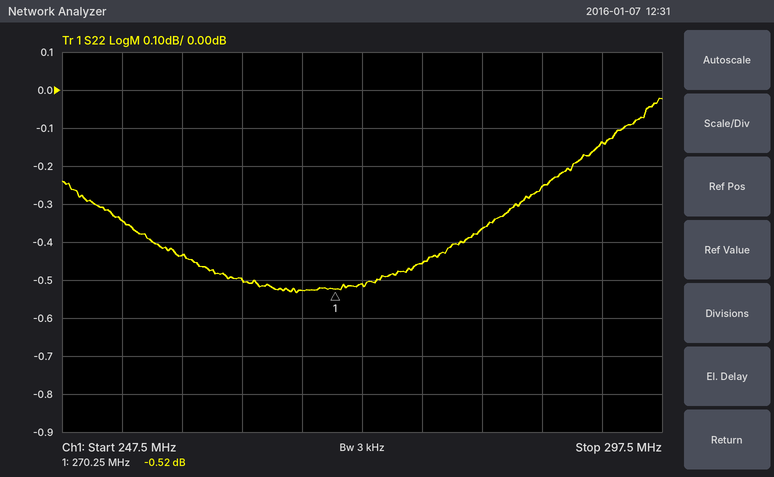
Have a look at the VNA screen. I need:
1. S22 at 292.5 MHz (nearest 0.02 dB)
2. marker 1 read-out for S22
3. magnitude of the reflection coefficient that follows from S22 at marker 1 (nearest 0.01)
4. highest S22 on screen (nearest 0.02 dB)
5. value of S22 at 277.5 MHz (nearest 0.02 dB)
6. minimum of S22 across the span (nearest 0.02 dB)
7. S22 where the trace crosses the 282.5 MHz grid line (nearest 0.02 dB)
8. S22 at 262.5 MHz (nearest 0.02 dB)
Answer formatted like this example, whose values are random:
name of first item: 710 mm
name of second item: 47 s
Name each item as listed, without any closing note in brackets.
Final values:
S22 at 292.5 MHz: -0.14 dB
marker 1 read-out for S22: -0.52 dB
magnitude of the reflection coefficient that follows from S22 at marker 1: 0.94
highest S22 on screen: -0.02 dB
value of S22 at 277.5 MHz: -0.46 dB
minimum of S22 across the span: -0.54 dB
S22 where the trace crosses the 282.5 MHz grid line: -0.36 dB
S22 at 262.5 MHz: -0.50 dB
